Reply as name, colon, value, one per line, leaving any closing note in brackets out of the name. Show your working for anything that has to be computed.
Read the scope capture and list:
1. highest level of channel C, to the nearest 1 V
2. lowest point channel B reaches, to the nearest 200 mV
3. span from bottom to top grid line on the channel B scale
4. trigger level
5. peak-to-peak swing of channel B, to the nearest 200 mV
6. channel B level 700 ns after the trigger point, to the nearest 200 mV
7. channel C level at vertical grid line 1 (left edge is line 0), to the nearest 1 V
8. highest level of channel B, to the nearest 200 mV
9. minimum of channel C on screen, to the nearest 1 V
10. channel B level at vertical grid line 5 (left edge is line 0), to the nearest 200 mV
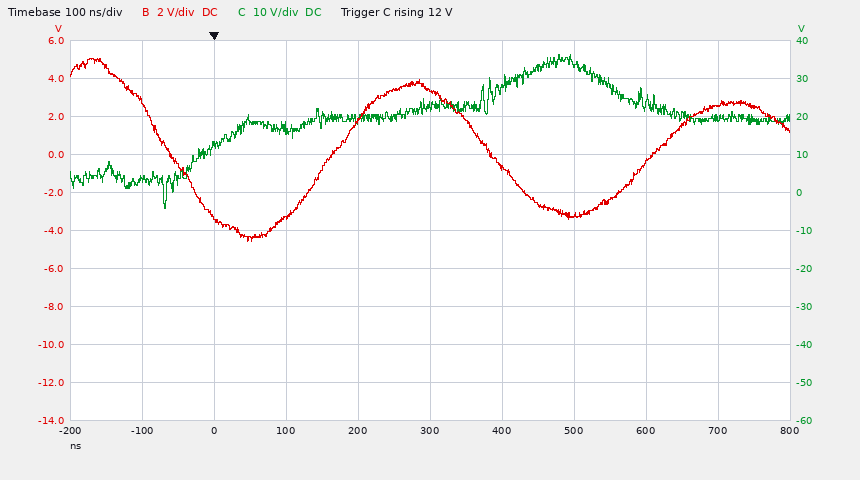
highest level of channel C, to the nearest 1 V: 36 V
lowest point channel B reaches, to the nearest 200 mV: -4.6 V
span from bottom to top grid line on the channel B scale: 20 V
trigger level: 12 V
peak-to-peak swing of channel B, to the nearest 200 mV: 5.0 V − (-4.6 V) = 9.6 V
channel B level 700 ns after the trigger point, to the nearest 200 mV: 2.6 V
channel C level at vertical grid line 1 (left edge is line 0), to the nearest 1 V: 4 V
highest level of channel B, to the nearest 200 mV: 5.0 V
minimum of channel C on screen, to the nearest 1 V: -4 V
channel B level at vertical grid line 5 (left edge is line 0), to the nearest 200 mV: 3.4 V
